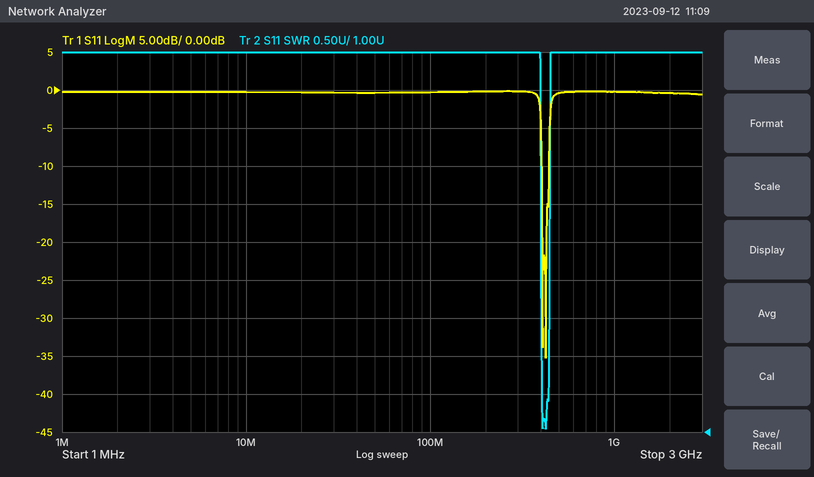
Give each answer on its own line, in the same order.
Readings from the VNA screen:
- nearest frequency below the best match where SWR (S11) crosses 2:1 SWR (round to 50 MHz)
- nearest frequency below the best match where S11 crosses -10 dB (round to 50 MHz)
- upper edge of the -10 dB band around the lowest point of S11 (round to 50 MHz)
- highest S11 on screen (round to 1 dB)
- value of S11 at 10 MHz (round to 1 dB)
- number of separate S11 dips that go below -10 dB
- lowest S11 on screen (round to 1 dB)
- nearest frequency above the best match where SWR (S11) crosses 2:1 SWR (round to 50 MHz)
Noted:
400 MHz
400 MHz
450 MHz
0 dB
0 dB
2
-35 dB
450 MHz
